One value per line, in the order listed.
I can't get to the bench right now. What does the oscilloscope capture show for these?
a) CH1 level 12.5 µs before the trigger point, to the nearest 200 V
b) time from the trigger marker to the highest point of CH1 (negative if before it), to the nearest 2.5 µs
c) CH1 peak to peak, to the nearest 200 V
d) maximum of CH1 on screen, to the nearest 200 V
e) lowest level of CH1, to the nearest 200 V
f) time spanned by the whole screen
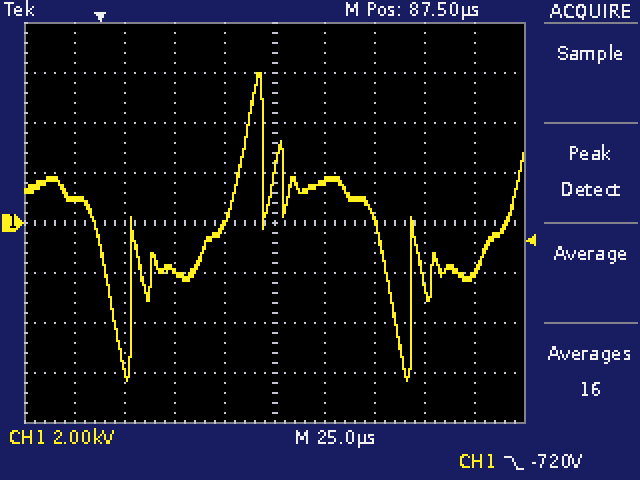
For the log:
1.0 kV
+80.0 µs
12.4 kV
6.0 kV
-6.4 kV
250 µs
